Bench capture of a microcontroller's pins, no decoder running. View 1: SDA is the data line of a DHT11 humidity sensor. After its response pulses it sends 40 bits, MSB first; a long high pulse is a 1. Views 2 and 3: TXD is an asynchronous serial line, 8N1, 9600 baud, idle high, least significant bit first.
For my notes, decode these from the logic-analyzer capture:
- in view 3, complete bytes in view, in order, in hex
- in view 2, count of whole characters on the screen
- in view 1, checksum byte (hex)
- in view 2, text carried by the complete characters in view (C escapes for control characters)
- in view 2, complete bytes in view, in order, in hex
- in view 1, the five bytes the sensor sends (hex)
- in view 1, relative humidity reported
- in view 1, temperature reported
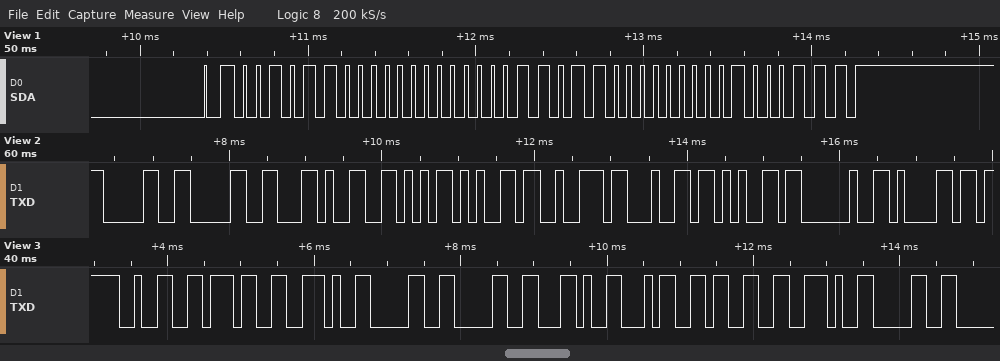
32 37 2E 30 30 2C 34 33 2E 30
10
0x47
"00,Verde a"
30 30 2C 56 65 72 64 65 20 61
2C 00 1B 00 47
44 %
27.0 °C
